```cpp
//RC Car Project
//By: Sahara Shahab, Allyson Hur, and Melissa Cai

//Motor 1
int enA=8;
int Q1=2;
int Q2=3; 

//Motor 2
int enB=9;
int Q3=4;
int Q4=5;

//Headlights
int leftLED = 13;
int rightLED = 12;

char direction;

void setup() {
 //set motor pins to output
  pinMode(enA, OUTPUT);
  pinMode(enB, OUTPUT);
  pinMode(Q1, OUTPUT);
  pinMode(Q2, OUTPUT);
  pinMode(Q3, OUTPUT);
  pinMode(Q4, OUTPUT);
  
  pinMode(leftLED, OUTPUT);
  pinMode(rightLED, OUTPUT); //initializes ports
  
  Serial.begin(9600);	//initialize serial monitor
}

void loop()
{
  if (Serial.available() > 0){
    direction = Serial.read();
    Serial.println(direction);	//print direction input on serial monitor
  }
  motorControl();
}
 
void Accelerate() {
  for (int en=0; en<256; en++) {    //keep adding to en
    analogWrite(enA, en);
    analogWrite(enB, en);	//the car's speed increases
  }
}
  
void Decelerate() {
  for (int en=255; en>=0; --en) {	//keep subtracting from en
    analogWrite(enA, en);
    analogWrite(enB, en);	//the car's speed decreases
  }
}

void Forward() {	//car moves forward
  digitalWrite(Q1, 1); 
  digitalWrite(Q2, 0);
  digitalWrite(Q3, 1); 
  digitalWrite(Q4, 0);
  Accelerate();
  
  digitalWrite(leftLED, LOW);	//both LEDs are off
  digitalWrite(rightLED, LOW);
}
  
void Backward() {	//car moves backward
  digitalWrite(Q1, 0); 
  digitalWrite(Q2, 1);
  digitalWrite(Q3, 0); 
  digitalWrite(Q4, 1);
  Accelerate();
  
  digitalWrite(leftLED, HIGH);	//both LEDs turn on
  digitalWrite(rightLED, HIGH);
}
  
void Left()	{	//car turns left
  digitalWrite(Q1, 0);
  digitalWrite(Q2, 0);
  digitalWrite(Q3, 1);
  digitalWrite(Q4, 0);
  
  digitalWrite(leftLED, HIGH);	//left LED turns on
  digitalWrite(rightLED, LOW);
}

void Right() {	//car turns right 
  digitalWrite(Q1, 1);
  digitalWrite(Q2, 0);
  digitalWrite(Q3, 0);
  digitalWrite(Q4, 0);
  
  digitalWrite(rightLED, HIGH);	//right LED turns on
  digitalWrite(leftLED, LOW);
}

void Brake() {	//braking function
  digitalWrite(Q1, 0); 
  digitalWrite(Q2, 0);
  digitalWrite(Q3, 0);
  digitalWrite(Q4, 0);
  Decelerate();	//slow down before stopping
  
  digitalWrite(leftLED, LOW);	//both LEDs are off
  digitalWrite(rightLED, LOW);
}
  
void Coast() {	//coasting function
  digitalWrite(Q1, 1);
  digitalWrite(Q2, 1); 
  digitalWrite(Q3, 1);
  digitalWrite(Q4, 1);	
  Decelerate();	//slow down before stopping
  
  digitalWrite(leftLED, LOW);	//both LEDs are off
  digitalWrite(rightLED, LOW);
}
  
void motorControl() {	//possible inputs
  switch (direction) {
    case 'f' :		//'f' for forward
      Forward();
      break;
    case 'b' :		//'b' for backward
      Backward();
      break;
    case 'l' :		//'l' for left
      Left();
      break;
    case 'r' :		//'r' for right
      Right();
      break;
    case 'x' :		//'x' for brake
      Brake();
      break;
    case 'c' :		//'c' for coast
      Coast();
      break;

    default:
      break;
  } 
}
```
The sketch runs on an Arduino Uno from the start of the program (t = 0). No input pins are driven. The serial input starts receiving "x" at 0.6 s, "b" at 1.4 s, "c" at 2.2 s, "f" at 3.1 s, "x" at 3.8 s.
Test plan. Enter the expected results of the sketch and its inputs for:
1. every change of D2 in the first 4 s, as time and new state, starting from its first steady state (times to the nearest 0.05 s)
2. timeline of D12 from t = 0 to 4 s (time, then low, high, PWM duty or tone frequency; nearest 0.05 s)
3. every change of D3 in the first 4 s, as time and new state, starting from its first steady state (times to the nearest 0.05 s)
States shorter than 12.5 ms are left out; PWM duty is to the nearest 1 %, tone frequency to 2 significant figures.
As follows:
0 s low; 2.2 s high; 3.8 s low
0 s low; 1.4 s high; 2.2 s low
0 s low; 1.4 s high; 3.1 s low
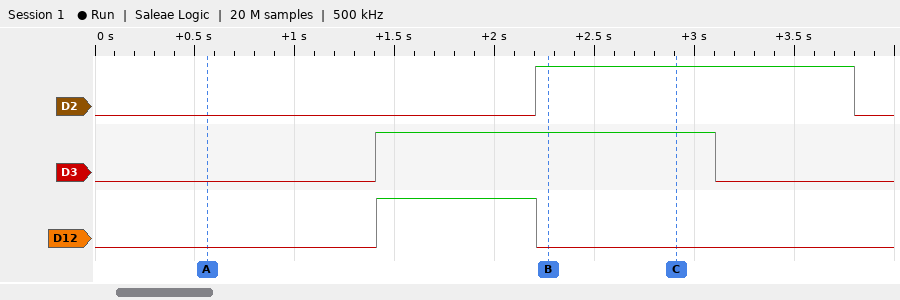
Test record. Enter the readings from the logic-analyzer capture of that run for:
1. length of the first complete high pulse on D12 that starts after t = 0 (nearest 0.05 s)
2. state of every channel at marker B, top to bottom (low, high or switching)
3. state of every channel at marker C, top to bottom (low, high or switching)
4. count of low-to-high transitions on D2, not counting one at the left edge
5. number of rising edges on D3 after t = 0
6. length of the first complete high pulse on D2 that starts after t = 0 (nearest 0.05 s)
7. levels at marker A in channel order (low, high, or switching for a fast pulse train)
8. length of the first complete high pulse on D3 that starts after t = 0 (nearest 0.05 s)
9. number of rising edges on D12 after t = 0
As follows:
0.80 s
D2 high, D3 high, D12 low
D2 high, D3 high, D12 low
1
1
1.60 s
D2 low, D3 low, D12 low
1.70 s
1
